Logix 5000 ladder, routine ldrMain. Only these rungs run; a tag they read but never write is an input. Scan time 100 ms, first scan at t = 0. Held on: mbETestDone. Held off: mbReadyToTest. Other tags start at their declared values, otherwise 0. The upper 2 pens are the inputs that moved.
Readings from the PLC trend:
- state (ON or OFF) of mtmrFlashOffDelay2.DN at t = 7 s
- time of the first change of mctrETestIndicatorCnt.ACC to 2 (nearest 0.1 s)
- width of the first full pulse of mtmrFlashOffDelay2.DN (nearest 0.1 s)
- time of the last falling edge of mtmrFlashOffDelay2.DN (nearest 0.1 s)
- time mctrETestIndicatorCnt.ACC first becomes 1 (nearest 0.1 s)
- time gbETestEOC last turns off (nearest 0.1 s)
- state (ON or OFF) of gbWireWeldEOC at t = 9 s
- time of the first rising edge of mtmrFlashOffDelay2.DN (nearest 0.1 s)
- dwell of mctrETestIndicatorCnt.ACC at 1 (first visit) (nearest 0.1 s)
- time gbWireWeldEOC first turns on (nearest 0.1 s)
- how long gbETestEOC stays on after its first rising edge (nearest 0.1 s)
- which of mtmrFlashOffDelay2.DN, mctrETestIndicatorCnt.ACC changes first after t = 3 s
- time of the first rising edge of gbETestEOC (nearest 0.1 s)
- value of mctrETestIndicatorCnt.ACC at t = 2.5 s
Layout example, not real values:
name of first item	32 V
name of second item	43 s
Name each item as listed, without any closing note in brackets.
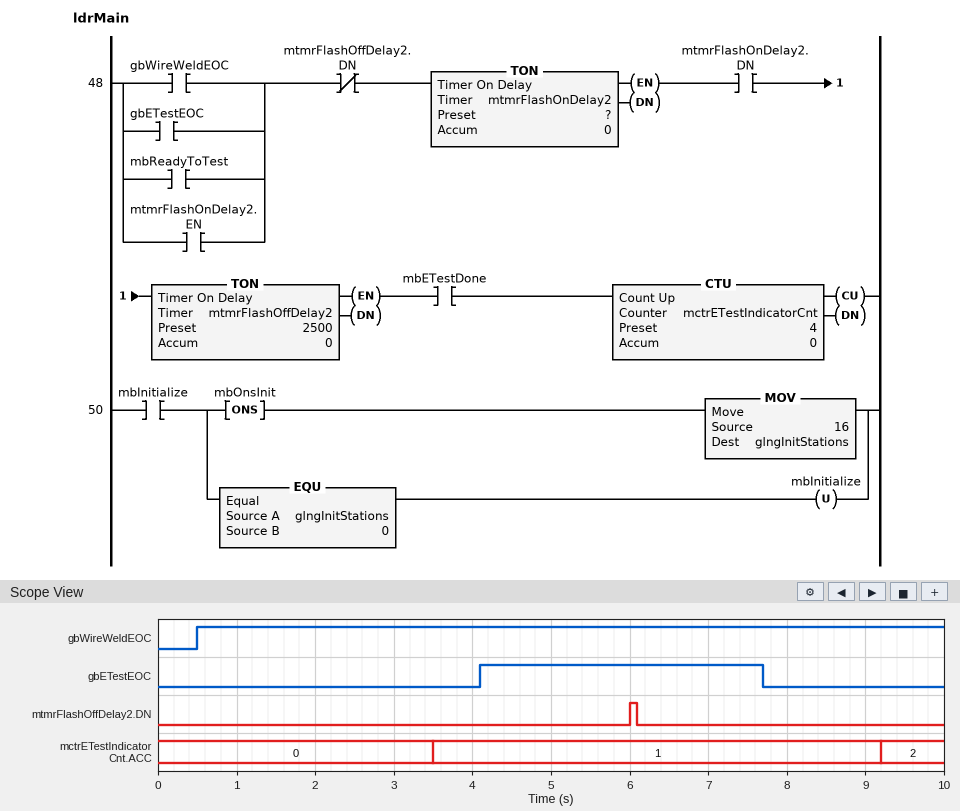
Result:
state (ON or OFF) of mtmrFlashOffDelay2.DN at t = 7 s	OFF
time of the first change of mctrETestIndicatorCnt.ACC to 2	9.2 s
width of the first full pulse of mtmrFlashOffDelay2.DN	0.1 s
time of the last falling edge of mtmrFlashOffDelay2.DN	6.1 s
time mctrETestIndicatorCnt.ACC first becomes 1	3.5 s
time gbETestEOC last turns off	7.7 s
state (ON or OFF) of gbWireWeldEOC at t = 9 s	ON
time of the first rising edge of mtmrFlashOffDelay2.DN	6.0 s
dwell of mctrETestIndicatorCnt.ACC at 1 (first visit)	5.7 s
time gbWireWeldEOC first turns on	0.5 s
how long gbETestEOC stays on after its first rising edge	3.6 s
which of mtmrFlashOffDelay2.DN, mctrETestIndicatorCnt.ACC changes first after t = 3 s	mctrETestIndicatorCnt.ACC
time of the first rising edge of gbETestEOC	4.1 s
value of mctrETestIndicatorCnt.ACC at t = 2.5 s	0
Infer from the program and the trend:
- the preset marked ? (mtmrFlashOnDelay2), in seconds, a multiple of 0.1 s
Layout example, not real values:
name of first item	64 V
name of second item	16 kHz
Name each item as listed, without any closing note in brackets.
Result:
the preset marked ? (mtmrFlashOnDelay2), in seconds, a multiple of 0.1 s	3.0 s
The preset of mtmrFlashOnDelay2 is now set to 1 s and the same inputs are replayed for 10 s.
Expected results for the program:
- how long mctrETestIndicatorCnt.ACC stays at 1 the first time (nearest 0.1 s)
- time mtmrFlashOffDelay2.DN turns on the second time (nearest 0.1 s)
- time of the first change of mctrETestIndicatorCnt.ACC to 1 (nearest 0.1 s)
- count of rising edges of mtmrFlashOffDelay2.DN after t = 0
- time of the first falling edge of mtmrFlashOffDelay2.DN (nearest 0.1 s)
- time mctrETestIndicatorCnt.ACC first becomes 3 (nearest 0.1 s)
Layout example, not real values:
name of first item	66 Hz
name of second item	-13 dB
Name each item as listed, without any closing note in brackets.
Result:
how long mctrETestIndicatorCnt.ACC stays at 1 the first time	3.7 s
time mtmrFlashOffDelay2.DN turns on the second time	7.7 s
time of the first change of mctrETestIndicatorCnt.ACC to 1	1.5 s
count of rising edges of mtmrFlashOffDelay2.DN after t = 0	2
time of the first falling edge of mtmrFlashOffDelay2.DN	4.1 s
time mctrETestIndicatorCnt.ACC first becomes 3	8.9 s
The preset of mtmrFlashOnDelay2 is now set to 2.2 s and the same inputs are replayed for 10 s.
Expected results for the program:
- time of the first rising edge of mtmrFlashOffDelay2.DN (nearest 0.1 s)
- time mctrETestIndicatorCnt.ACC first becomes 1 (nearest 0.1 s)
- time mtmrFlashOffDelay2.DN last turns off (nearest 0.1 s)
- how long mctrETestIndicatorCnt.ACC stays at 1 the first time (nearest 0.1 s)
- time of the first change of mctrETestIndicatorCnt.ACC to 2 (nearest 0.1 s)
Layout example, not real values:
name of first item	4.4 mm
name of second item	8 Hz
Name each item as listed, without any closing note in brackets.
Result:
time of the first rising edge of mtmrFlashOffDelay2.DN	5.2 s
time mctrETestIndicatorCnt.ACC first becomes 1	2.7 s
time mtmrFlashOffDelay2.DN last turns off	5.3 s
how long mctrETestIndicatorCnt.ACC stays at 1 the first time	4.9 s
time of the first change of mctrETestIndicatorCnt.ACC to 2	7.6 s
